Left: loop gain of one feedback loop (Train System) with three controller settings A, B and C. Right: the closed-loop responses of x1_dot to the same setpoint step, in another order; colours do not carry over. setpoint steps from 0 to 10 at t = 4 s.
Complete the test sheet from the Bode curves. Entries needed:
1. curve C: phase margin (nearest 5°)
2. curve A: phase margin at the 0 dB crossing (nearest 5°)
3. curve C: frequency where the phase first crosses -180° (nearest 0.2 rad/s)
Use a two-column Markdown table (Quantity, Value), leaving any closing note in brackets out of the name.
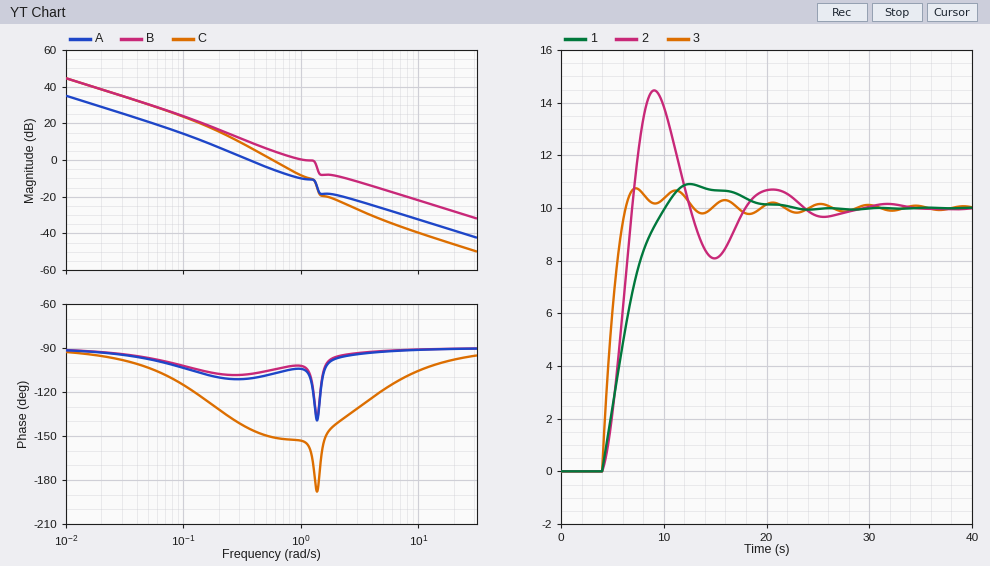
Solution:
| Quantity | Value |
|---|---|
| curve C: phase margin | 30° |
| curve A: phase margin at the 0 dB crossing | 70° |
| curve C: frequency where the phase first crosses -180° | 1.4 rad/s |
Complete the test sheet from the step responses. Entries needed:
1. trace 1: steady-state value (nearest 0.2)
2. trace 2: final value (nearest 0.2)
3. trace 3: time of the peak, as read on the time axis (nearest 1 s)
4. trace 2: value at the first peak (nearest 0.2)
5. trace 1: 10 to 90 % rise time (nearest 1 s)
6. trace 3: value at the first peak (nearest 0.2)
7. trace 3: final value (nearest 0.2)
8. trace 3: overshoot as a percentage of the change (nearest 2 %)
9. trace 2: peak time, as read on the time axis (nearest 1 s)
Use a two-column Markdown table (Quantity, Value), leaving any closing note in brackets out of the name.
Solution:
| Quantity | Value |
|---|---|
| trace 1: steady-state value | 10.0 |
| trace 2: final value | 10.0 |
| trace 3: time of the peak, as read on the time axis | 7 s |
| trace 2: value at the first peak | 14.4 |
| trace 1: 10 to 90 % rise time | 4 s |
| trace 3: value at the first peak | 10.8 |
| trace 3: final value | 10.0 |
| trace 3: overshoot as a percentage of the change | 8 % |
| trace 2: peak time, as read on the time axis | 9 s |
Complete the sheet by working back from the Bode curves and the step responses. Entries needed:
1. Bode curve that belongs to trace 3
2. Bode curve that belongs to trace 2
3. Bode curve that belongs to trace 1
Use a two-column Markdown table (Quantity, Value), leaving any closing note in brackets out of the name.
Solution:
| Quantity | Value |
|---|---|
| Bode curve that belongs to trace 3 | B |
| Bode curve that belongs to trace 2 | C |
| Bode curve that belongs to trace 1 | A |
